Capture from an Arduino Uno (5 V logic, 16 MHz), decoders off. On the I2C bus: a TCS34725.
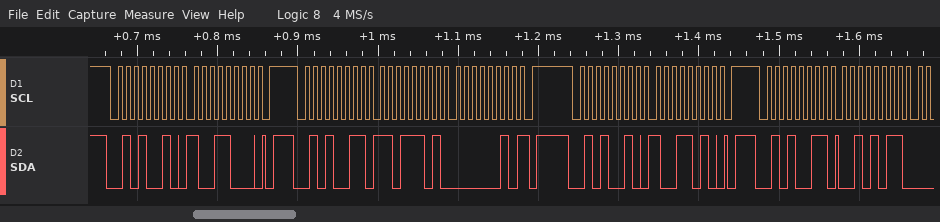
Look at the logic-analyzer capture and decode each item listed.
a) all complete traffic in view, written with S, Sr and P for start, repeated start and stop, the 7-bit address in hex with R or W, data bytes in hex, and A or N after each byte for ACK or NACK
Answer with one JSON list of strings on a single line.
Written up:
["S 29W A 98 A P S 29R A DD A 02 N P S 29W A 9A A P S 29R A 2B A"]
